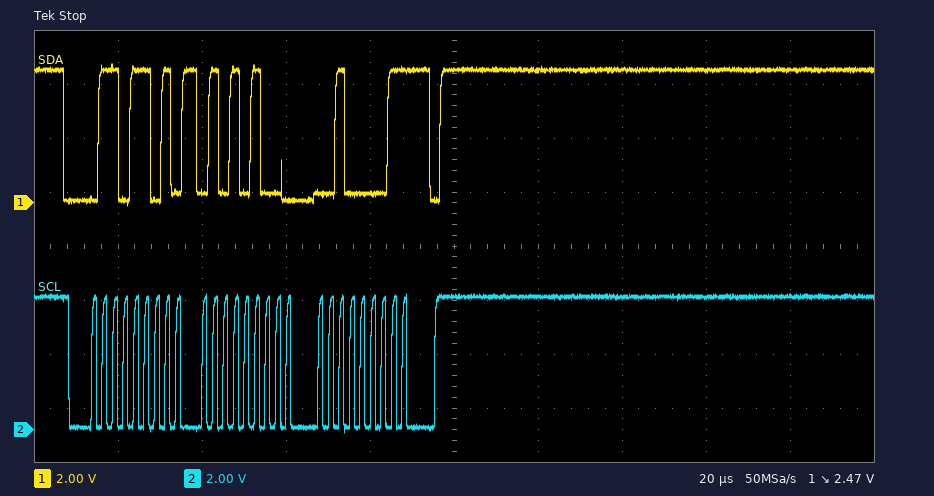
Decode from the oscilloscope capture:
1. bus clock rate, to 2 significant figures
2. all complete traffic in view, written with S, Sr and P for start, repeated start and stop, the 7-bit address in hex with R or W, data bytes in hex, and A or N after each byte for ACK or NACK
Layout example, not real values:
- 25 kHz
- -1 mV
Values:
- 400 kHz
- S 36R A 54 A 21 N P
